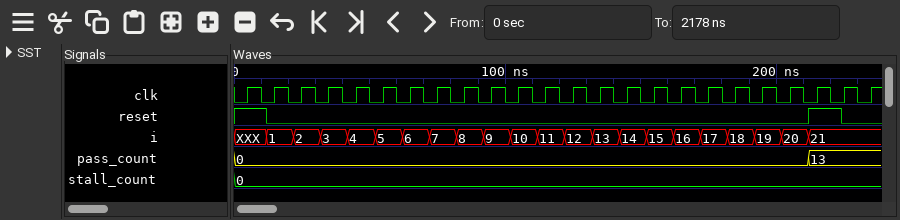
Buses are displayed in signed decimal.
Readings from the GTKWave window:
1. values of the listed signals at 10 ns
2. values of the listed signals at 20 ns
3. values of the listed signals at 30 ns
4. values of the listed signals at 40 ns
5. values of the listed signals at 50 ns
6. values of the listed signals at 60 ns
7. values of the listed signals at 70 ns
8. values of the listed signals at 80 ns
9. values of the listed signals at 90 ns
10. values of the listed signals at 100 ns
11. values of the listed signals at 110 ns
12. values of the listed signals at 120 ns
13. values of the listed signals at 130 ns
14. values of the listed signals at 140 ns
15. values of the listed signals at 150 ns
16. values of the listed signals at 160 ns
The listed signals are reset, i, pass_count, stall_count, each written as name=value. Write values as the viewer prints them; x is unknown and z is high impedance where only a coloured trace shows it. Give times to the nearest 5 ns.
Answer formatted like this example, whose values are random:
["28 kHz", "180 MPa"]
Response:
["reset=1, i=XXX, pass_count=0, stall_count=0", "reset=0, i=1, pass_count=0, stall_count=0", "reset=0, i=2, pass_count=0, stall_count=0", "reset=0, i=3, pass_count=0, stall_count=0", "reset=0, i=4, pass_count=0, stall_count=0", "reset=0, i=5, pass_count=0, stall_count=0", "reset=0, i=6, pass_count=0, stall_count=0", "reset=0, i=7, pass_count=0, stall_count=0", "reset=0, i=8, pass_count=0, stall_count=0", "reset=0, i=9, pass_count=0, stall_count=0", "reset=0, i=10, pass_count=0, stall_count=0", "reset=0, i=11, pass_count=0, stall_count=0", "reset=0, i=12, pass_count=0, stall_count=0", "reset=0, i=13, pass_count=0, stall_count=0", "reset=0, i=14, pass_count=0, stall_count=0", "reset=0, i=15, pass_count=0, stall_count=0"]
